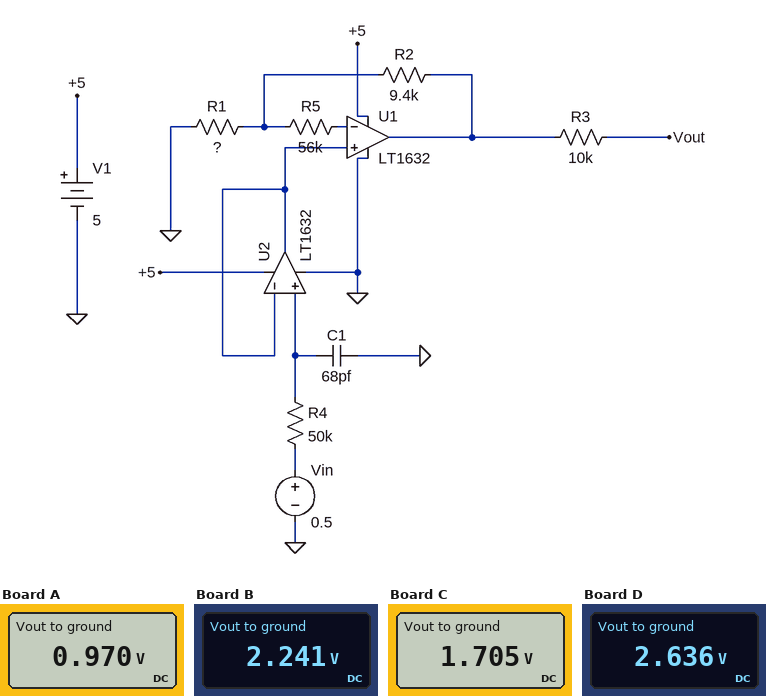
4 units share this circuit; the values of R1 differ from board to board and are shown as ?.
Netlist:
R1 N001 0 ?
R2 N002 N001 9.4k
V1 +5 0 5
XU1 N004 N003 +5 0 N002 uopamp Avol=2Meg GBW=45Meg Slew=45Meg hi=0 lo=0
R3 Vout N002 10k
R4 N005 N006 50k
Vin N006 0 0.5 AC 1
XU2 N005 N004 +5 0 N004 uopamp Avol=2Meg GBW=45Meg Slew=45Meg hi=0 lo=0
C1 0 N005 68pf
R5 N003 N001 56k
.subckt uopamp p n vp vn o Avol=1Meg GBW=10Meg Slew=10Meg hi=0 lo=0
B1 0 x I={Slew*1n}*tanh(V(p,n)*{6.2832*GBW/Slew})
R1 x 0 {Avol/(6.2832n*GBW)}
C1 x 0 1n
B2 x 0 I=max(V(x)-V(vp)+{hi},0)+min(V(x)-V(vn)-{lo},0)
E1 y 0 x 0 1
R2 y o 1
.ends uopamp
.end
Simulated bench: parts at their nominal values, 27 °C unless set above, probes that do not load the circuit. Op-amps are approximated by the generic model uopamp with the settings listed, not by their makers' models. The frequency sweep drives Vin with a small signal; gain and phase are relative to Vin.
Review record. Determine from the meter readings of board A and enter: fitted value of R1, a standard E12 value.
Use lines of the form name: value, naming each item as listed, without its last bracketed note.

fitted value of R1, a standard E12 value: 10 kΩ
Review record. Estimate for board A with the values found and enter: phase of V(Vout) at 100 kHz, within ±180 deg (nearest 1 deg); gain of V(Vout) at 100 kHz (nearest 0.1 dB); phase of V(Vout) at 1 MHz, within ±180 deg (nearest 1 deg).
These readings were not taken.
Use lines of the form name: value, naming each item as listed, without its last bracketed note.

phase of V(Vout) at 100 kHz, within ±180 deg: -65 deg
gain of V(Vout) at 100 kHz: -1.7 dB
phase of V(Vout) at 1 MHz, within ±180 deg: -91 deg
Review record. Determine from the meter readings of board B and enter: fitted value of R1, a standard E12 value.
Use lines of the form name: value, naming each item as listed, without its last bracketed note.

fitted value of R1, a standard E12 value: 2.7 kΩ
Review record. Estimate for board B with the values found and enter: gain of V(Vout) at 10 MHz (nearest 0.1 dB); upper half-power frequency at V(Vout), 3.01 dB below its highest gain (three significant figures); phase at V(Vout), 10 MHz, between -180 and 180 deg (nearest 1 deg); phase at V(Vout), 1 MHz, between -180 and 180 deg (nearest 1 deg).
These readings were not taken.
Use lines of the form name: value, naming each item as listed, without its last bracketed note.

gain of V(Vout) at 10 MHz: -36.8 dB
upper half-power frequency at V(Vout), 3.01 dB below its highest gain: 46.8 kHz
phase at V(Vout), 10 MHz, between -180 and 180 deg: -147 deg
phase at V(Vout), 1 MHz, between -180 and 180 deg: -94 deg
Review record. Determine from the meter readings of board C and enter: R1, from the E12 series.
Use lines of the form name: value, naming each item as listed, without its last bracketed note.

R1, from the E12 series: 3.9 kΩ
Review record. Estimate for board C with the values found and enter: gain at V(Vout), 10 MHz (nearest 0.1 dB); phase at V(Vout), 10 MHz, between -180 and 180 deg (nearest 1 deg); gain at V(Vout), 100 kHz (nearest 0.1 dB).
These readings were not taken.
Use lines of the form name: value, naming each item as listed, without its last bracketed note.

gain at V(Vout), 10 MHz: -38.1 dB
phase at V(Vout), 10 MHz, between -180 and 180 deg: -139 deg
gain at V(Vout), 100 kHz: 3.2 dB
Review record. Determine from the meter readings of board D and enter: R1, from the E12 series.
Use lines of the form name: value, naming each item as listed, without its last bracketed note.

R1, from the E12 series: 2.2 kΩ
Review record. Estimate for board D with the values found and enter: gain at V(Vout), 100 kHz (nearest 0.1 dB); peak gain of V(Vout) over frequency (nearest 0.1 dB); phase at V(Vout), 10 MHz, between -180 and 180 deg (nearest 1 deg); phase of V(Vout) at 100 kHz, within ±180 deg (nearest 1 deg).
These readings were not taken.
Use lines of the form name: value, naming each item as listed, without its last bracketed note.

gain at V(Vout), 100 kHz: 7.0 dB
peak gain of V(Vout) over frequency: 14.4 dB
phase at V(Vout), 10 MHz, between -180 and 180 deg: -152 deg
phase of V(Vout) at 100 kHz, within ±180 deg: -66 deg
